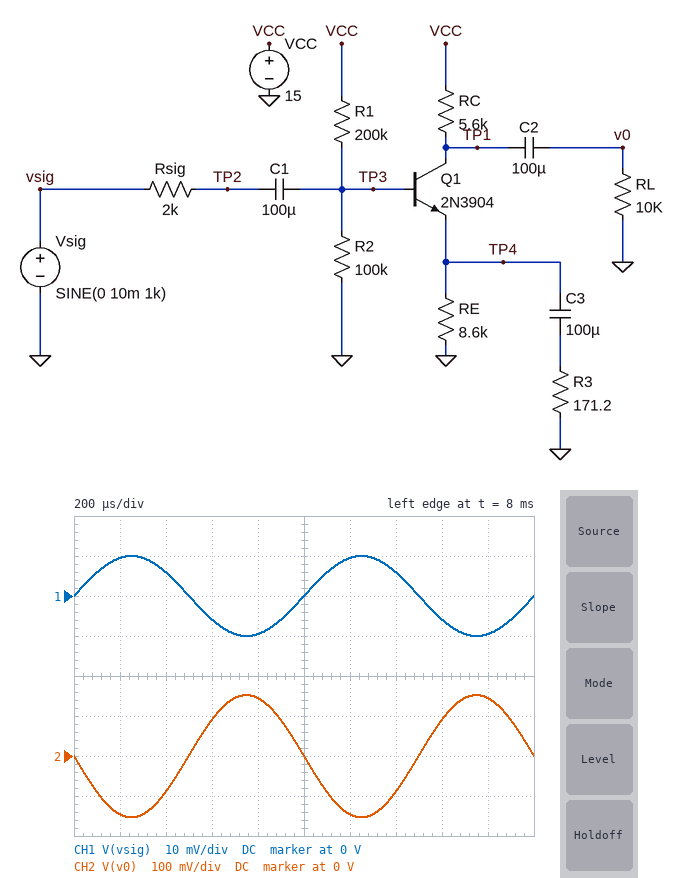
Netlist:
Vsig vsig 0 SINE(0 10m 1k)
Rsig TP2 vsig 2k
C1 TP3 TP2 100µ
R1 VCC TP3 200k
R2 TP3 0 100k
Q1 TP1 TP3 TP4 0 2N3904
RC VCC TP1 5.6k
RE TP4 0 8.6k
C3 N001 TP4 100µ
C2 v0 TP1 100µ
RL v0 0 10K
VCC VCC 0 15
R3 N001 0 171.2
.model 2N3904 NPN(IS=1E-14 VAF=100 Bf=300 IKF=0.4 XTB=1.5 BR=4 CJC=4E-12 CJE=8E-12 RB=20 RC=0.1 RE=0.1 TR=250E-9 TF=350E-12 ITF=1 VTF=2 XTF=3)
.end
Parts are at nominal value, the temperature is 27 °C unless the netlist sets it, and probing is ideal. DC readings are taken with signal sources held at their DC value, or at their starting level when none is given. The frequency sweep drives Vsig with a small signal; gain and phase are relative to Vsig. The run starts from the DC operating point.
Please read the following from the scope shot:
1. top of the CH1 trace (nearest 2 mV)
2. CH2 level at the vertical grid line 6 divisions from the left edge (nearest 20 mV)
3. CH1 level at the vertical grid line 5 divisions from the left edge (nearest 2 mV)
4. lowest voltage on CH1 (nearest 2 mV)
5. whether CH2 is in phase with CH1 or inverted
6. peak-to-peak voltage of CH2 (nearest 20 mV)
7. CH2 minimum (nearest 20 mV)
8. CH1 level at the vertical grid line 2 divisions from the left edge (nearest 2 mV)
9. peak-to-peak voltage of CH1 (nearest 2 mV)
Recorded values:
10 mV
-140 mV
0 V
-10 mV
inverted
300 mV
-160 mV
6 mV
20 mV
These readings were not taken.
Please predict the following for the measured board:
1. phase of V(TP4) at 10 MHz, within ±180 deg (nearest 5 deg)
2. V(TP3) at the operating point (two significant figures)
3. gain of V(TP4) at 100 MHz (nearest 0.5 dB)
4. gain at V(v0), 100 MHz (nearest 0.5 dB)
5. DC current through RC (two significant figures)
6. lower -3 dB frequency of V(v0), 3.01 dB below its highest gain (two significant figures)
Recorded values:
-55 deg
4.9 V
-23.5 dB
-9.5 dB
490 µA
6.9 Hz
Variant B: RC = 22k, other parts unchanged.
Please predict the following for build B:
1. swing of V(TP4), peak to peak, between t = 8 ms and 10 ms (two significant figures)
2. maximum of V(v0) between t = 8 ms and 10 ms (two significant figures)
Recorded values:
7.0 mV
210 mV
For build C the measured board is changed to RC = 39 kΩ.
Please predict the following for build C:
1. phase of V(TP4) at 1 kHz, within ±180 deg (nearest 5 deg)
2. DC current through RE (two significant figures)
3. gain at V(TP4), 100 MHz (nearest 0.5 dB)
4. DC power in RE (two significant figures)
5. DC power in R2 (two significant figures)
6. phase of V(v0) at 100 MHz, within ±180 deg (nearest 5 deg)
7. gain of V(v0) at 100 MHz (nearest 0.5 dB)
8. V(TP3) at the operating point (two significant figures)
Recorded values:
0 deg
330 µA
-22.5 dB
950 µW
120 µW
-5 deg
-20.5 dB
3.5 V
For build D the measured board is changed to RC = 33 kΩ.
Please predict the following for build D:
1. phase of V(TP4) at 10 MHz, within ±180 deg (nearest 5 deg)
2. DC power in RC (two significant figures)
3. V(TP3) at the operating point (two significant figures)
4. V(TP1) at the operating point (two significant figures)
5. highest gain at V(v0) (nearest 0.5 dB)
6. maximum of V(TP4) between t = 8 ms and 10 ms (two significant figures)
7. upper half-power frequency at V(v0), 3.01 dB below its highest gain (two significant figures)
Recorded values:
0 deg
4.2 mW
3.8 V
3.3 V
-7.0 dB
3.2 V
190 kHz
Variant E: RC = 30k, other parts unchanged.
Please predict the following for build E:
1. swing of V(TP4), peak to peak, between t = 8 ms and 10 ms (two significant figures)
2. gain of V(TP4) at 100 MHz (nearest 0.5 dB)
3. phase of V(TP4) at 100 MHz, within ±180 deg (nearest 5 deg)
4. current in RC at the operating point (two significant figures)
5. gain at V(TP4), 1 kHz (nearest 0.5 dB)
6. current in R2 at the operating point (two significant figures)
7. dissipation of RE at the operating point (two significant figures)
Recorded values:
1.6 mV
-22.5 dB
0 deg
380 µA
-22.0 dB
41 µA
1.4 mW
